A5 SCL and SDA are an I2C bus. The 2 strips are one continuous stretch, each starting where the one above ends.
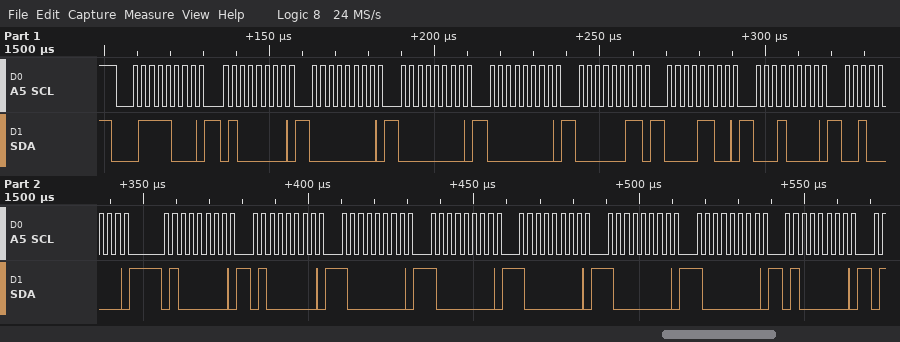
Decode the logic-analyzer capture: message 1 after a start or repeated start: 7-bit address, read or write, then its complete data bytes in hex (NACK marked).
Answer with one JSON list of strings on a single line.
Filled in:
["0x3C write: 40 00 00 00 03 0C 10 20 40 40 80 80 80 80 80 40"]
